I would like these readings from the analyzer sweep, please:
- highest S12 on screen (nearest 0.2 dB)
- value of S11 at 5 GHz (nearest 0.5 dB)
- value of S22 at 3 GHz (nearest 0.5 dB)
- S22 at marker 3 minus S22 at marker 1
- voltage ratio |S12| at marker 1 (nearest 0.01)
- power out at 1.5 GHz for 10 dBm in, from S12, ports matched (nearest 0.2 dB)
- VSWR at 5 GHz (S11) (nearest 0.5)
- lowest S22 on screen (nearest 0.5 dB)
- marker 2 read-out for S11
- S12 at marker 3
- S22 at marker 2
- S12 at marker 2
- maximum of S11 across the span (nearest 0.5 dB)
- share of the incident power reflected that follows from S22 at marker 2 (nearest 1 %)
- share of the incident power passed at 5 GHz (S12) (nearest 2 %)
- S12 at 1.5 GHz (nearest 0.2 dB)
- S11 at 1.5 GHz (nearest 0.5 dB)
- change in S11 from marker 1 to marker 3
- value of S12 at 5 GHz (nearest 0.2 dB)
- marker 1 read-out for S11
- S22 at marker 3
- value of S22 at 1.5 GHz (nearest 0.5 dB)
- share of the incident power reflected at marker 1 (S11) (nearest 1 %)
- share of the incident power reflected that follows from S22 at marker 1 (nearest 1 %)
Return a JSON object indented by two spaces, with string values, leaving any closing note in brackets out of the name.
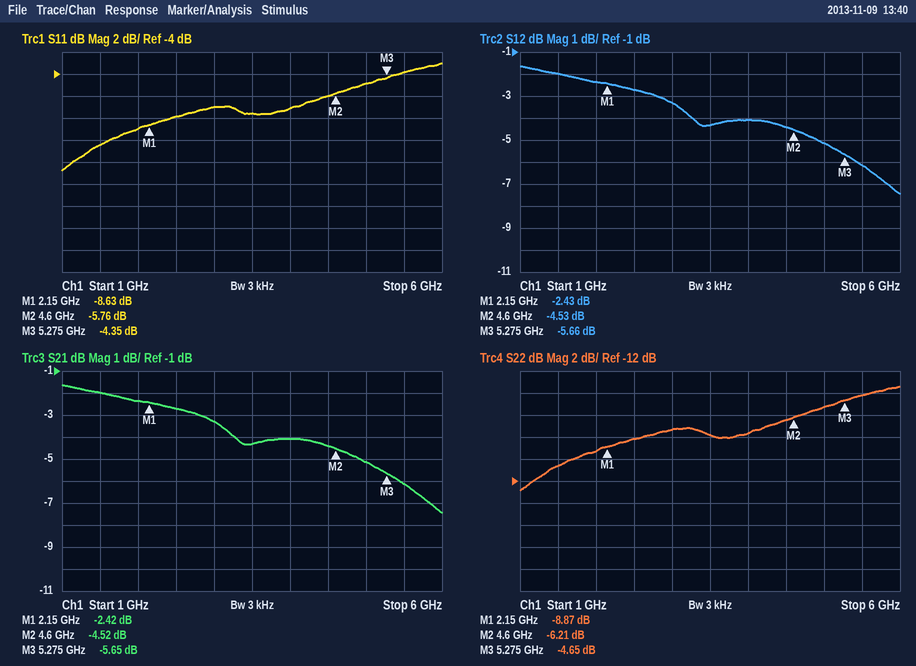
{
  "highest S12 on screen": "-1.6 dB",
  "value of S11 at 5 GHz": "-5.0 dB",
  "value of S22 at 3 GHz": "-7.5 dB",
  "S22 at marker 3 minus S22 at marker 1": "4.22 dB",
  "voltage ratio |S12| at marker 1": "0.76",
  "power out at 1.5 GHz for 10 dBm in, from S12, ports matched": "8.0 dBm",
  "VSWR at 5 GHz (S11)": "3.5",
  "lowest S22 on screen": "-13.0 dB",
  "marker 2 read-out for S11": "-5.76 dB",
  "S12 at marker 3": "-5.66 dB",
  "S22 at marker 2": "-6.21 dB",
  "S12 at marker 2": "-4.53 dB",
  "maximum of S11 across the span": "-3.0 dB",
  "share of the incident power reflected that follows from S22 at marker 2": "24 %",
  "share of the incident power passed at 5 GHz (S12)": "30 %",
  "S12 at 1.5 GHz": "-2.0 dB",
  "S11 at 1.5 GHz": "-10.5 dB",
  "change in S11 from marker 1 to marker 3": "4.28 dB",
  "value of S12 at 5 GHz": "-5.2 dB",
  "marker 1 read-out for S11": "-8.63 dB",
  "S22 at marker 3": "-4.65 dB",
  "value of S22 at 1.5 GHz": "-10.5 dB",
  "share of the incident power reflected at marker 1 (S11)": "14 %",
  "share of the incident power reflected that follows from S22 at marker 1": "13 %"
}
